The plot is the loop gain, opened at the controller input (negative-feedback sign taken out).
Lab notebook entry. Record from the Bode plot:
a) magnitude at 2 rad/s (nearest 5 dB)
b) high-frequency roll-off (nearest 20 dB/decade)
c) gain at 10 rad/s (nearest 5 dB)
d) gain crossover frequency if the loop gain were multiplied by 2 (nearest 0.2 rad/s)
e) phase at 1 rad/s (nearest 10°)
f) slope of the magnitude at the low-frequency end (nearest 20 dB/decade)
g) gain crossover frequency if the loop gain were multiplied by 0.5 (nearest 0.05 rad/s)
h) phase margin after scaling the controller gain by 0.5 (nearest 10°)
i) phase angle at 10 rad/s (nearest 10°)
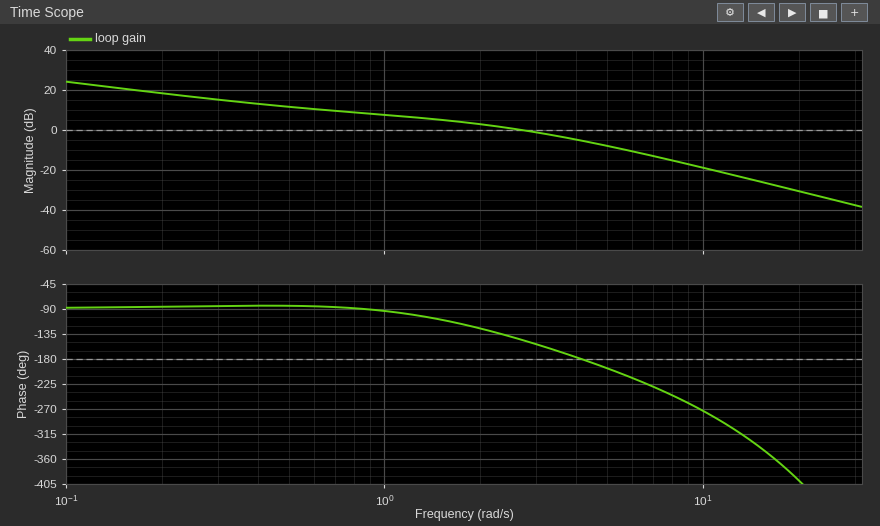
5 dB
-40 dB/decade
-20 dB
4.4 rad/s
-90°
-20 dB/decade
1.30 rad/s
80°
-270°
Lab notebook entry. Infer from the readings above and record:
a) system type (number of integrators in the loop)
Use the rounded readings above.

1
